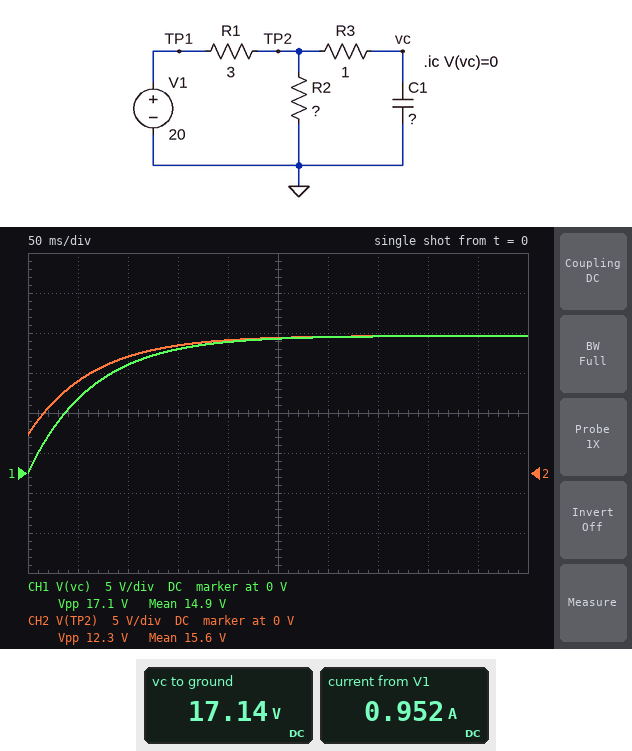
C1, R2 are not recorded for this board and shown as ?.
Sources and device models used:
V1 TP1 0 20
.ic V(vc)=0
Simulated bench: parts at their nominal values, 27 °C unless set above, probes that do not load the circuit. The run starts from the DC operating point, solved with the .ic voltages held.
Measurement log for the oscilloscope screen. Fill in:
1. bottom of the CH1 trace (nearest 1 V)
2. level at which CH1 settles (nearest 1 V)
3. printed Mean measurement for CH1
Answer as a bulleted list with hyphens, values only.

- 0 V
- 17 V
- 14.9 V
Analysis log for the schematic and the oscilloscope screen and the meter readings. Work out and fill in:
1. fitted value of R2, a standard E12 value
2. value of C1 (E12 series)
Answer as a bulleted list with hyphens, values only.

- 18 Ω
- 18 mF
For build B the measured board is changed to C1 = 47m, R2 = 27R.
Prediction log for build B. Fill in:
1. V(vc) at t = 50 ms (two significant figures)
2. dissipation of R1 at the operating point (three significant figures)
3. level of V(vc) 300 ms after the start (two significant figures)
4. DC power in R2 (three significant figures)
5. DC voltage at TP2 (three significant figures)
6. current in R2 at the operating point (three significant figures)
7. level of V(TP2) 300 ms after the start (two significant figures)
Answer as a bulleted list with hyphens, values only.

- 4.5 V
- 1.33 W
- 15 V
- 12.0 W
- 18.0 V
- 667 mA
- 16 V
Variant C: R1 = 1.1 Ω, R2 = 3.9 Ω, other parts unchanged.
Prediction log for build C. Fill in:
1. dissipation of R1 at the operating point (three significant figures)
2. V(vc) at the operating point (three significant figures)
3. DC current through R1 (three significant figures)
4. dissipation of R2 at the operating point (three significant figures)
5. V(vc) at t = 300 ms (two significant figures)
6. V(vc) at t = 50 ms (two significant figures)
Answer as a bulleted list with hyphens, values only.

- 17.6 W
- 15.6 V
- 4.00 A
- 62.4 W
- 16 V
- 12 V
